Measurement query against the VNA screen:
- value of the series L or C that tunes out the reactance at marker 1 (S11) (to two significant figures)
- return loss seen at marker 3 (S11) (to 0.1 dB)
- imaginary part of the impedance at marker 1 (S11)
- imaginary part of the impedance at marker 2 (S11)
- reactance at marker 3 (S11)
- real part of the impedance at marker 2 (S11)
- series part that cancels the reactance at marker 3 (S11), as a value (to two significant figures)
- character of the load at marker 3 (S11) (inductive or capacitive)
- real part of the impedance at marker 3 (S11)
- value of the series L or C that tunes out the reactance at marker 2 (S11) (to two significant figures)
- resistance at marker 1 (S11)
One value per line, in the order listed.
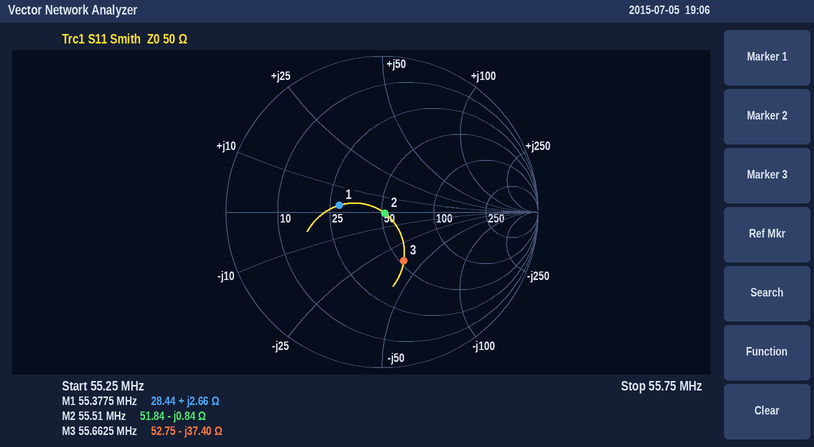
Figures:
1.1 nF
9.3 dB
+2.66 Ω
-0.84 Ω
-37.40 Ω
51.84 Ω
110 nH
capacitive
52.75 Ω
2.4 nH
28.44 Ω
